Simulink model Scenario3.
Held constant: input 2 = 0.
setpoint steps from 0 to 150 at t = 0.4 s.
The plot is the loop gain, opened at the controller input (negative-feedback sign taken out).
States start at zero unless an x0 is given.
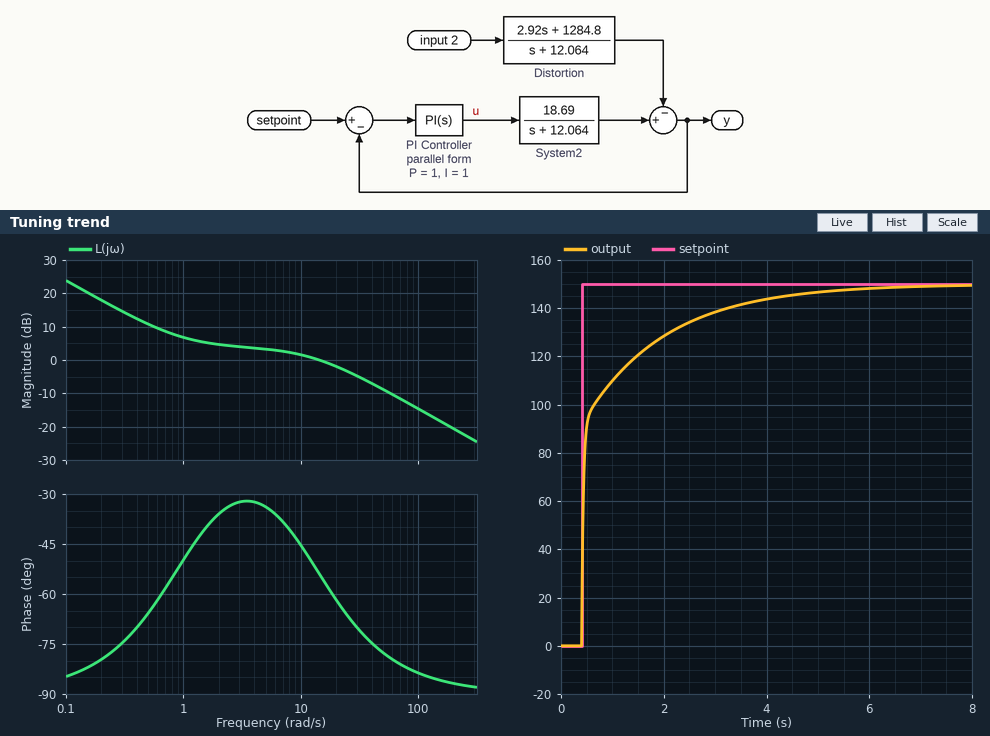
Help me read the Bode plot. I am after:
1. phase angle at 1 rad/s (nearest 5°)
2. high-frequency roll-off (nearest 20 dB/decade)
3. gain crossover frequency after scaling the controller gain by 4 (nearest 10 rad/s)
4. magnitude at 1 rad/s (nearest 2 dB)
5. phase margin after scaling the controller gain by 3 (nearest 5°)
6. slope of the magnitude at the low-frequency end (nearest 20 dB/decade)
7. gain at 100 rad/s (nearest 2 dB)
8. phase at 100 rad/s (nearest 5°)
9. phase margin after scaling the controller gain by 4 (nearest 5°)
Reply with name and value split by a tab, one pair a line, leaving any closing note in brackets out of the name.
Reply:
phase angle at 1 rad/s	-50°
high-frequency roll-off	-20 dB/decade
gain crossover frequency after scaling the controller gain by 4	70 rad/s
magnitude at 1 rad/s	6 dB
phase margin after scaling the controller gain by 3	100°
slope of the magnitude at the low-frequency end	-20 dB/decade
gain at 100 rad/s	-14 dB
phase at 100 rad/s	-85°
phase margin after scaling the controller gain by 4	100°
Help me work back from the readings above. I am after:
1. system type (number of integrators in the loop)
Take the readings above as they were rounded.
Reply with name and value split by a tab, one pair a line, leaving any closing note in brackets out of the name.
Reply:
system type	1
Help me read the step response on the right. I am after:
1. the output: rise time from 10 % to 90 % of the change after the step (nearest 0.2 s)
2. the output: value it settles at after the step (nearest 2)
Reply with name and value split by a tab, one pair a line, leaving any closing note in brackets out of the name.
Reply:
the output: rise time from 10 % to 90 % of the change after the step	2.2 s
the output: value it settles at after the step	150
